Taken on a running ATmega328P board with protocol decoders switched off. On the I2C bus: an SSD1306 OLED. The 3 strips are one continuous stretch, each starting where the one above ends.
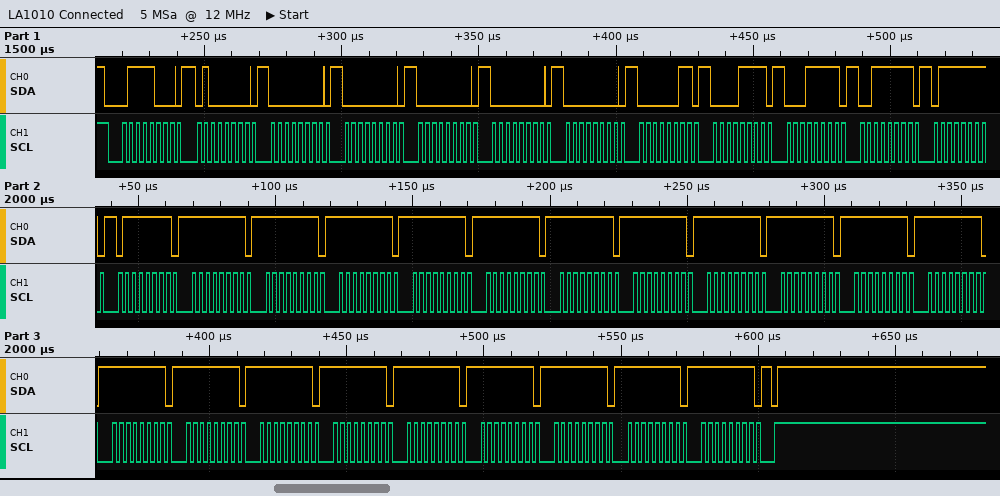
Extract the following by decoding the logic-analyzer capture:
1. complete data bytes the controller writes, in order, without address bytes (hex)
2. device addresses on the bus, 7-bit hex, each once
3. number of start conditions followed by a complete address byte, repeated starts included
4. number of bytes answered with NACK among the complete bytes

40 00 00 00 00 00 03 0F 1F 3F 7F 7F FF FF FF FF FF FF FF FF FF FF FF FF FF FF FF FF FF FF FF FF
0x3C
1
0
